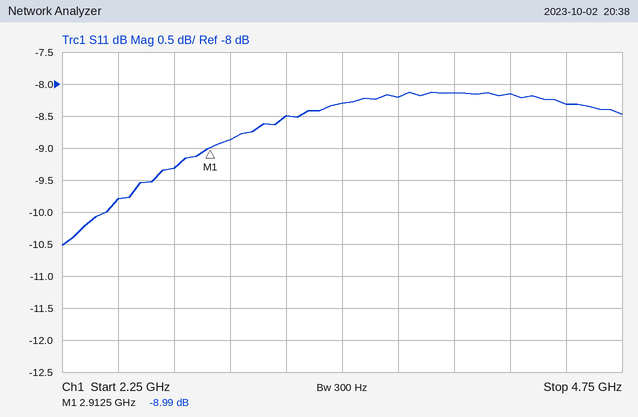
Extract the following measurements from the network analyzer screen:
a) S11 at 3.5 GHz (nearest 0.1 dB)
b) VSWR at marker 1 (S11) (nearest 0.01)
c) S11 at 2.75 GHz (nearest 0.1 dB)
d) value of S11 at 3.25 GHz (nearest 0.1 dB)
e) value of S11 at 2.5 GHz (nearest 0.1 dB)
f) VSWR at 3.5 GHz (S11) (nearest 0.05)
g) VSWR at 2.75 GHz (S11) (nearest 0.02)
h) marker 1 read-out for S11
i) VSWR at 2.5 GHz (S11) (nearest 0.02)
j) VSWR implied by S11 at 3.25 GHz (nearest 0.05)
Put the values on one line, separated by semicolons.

-8.3 dB; 2.10; -9.3 dB; -8.5 dB; -9.8 dB; 2.25; 2.04; -8.99 dB; 1.96; 2.20
